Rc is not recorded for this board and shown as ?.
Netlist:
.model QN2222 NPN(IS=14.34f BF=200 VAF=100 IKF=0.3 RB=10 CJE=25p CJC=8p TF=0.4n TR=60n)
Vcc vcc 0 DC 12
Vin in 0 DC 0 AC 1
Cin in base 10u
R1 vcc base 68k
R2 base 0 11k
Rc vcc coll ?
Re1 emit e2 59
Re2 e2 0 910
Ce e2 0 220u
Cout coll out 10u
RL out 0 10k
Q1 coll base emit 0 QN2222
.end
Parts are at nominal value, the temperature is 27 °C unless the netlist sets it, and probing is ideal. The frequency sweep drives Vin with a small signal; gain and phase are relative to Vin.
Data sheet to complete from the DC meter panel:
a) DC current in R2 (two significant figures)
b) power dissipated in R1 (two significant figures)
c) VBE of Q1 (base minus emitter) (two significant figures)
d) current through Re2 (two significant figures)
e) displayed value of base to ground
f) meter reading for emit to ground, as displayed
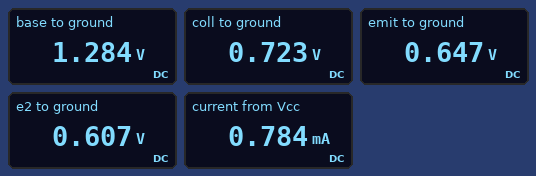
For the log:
120 µA
1.7 mW
640 mV
670 µA
1.284 V
0.647 V
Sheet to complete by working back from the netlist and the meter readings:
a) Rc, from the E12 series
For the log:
18 kΩ
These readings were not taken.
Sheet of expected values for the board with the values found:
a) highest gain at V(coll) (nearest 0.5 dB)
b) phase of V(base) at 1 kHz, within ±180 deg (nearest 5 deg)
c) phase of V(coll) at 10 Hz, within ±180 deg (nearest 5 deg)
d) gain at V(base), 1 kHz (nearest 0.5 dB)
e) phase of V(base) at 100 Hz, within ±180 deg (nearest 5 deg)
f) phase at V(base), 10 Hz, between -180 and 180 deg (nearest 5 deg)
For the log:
11.0 dB
5 deg
-85 deg
0 dB
45 deg
60 deg
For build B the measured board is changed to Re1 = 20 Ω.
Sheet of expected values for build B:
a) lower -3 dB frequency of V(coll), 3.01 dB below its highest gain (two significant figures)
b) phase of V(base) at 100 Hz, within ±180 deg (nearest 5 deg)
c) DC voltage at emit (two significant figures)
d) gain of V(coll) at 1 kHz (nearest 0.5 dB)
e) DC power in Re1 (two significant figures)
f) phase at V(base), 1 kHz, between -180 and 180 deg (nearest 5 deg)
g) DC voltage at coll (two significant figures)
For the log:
160 Hz
55 deg
620 mV
14.0 dB
9.0 µW
10 deg
700 mV
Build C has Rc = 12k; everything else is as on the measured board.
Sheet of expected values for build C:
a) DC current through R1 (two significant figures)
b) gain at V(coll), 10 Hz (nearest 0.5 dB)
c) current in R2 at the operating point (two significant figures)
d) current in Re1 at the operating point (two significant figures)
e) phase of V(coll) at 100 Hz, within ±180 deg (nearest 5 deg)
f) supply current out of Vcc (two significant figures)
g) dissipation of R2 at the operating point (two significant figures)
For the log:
150 µA
4.0 dB
140 µA
930 µA
-135 deg
1.1 mA
220 µW
